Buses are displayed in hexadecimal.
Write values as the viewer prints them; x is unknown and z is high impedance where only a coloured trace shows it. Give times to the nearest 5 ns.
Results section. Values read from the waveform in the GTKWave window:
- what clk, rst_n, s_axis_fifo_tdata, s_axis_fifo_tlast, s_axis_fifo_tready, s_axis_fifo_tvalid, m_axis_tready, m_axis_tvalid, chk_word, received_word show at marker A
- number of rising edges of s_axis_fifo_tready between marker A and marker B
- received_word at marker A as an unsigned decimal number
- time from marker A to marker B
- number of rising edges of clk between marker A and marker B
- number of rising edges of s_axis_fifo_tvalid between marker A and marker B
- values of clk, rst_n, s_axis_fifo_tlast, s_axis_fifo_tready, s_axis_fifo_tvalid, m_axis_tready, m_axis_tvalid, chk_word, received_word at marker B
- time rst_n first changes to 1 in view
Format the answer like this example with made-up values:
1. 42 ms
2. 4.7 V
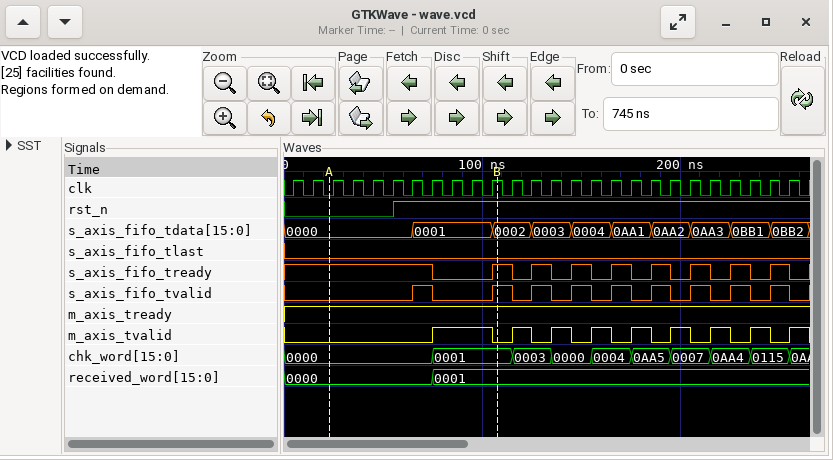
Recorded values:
1. clk=0, rst_n=0, s_axis_fifo_tdata=0000, s_axis_fifo_tlast=0, s_axis_fifo_tready=1, s_axis_fifo_tvalid=0, m_axis_tready=1, m_axis_tvalid=0, chk_word=0000, received_word=0000
2. 1
3. 0
4. 85 ns
5. 9
6. 2
7. clk=1, rst_n=1, s_axis_fifo_tlast=0, s_axis_fifo_tready=1, s_axis_fifo_tvalid=1, m_axis_tready=1, m_axis_tvalid=0, chk_word=0001, received_word=0001
8. 55 ns
